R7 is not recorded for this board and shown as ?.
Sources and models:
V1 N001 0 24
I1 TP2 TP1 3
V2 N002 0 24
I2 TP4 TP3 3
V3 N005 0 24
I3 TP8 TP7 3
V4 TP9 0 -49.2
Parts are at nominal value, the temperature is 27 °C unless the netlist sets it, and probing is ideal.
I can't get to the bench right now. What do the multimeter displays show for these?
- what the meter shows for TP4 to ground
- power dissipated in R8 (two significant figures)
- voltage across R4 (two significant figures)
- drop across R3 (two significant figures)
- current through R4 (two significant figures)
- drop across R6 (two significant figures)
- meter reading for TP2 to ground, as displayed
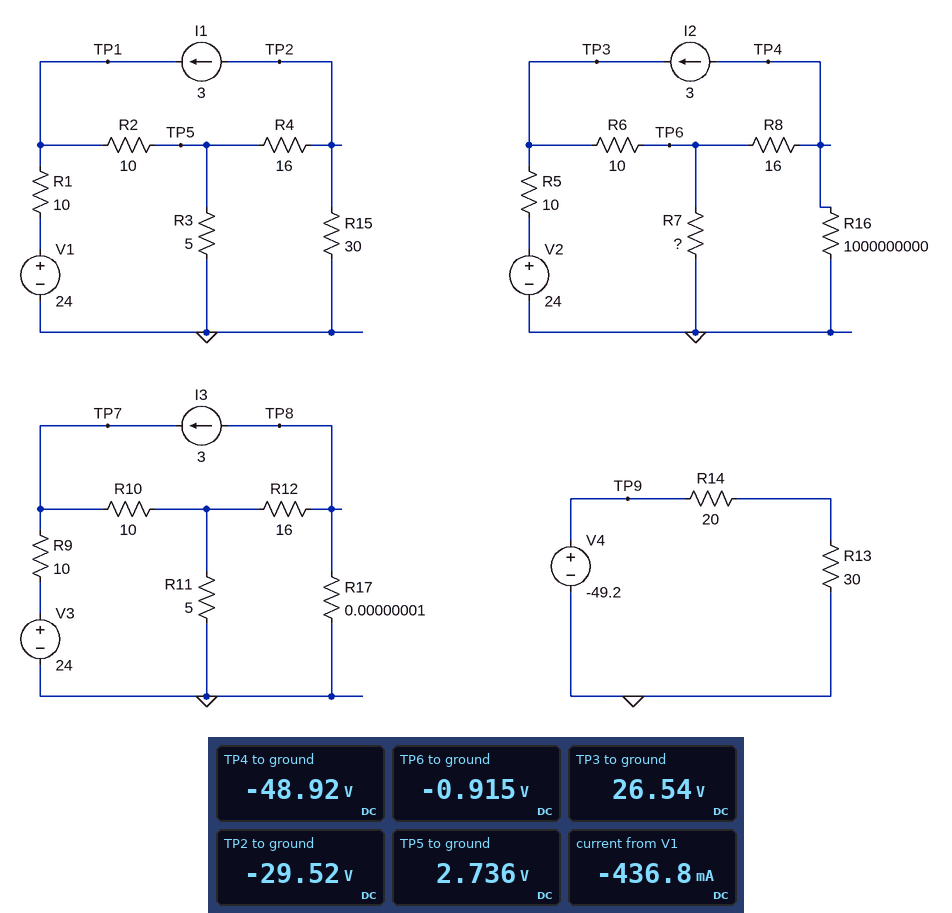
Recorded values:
-48.92 V
140 W
32 V
2.7 V
2.0 A
27 V
-29.52 V
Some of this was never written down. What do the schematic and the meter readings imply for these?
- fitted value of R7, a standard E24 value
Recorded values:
3.6 Ω
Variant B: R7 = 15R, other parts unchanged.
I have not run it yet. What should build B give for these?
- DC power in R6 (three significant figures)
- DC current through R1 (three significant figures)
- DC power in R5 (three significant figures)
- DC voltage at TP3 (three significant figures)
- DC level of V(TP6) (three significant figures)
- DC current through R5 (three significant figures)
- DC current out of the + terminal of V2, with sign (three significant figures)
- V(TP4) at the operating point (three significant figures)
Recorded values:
80.0 W
437 mA
294 mW
25.7 V
-2.57 V
171 mA
-171 mA
-50.6 V
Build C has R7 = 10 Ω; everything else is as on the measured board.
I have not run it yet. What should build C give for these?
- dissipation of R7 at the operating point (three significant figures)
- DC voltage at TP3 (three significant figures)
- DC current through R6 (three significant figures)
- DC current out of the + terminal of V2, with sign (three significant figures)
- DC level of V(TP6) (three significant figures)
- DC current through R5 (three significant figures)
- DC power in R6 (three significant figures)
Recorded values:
400 mW
26.0 V
2.80 A
-200 mA
-2.00 V
200 mA
78.4 W
